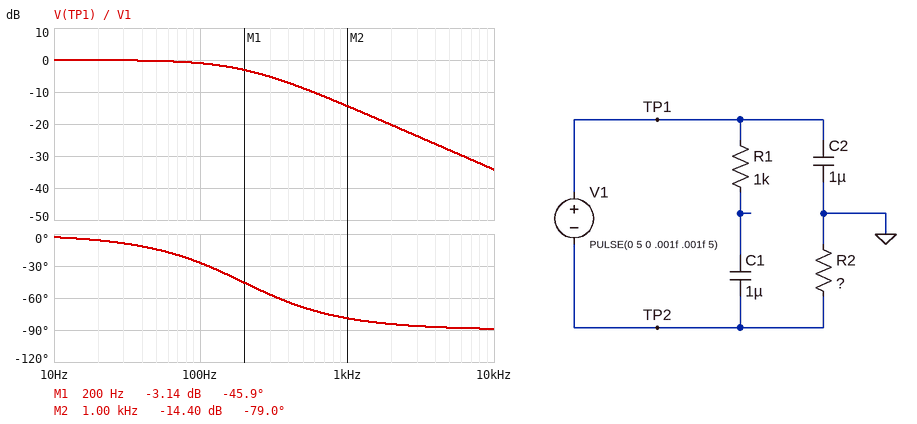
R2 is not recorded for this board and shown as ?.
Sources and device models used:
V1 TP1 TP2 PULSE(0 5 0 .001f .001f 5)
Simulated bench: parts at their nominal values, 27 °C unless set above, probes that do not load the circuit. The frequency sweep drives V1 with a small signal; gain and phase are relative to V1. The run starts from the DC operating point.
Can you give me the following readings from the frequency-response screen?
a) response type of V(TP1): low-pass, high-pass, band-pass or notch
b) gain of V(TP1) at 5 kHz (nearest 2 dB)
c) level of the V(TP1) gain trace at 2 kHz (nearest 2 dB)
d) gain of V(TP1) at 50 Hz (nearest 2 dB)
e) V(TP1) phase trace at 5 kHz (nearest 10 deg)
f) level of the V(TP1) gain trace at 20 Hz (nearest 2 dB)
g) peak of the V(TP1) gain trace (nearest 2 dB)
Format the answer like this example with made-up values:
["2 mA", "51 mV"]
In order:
["low-pass", "-28 dB", "-20 dB", "0 dB", "-90 deg", "0 dB", "0 dB"]
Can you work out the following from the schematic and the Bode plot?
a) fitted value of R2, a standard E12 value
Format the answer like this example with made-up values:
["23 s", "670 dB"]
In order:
["820 Ω"]
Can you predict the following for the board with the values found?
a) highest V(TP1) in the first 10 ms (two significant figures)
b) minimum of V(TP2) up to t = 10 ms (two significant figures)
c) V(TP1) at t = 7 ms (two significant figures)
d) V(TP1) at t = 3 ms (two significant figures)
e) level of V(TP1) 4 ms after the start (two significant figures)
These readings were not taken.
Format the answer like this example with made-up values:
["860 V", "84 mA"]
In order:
["5.0 V", "-5.0 V", "5.0 V", "4.9 V", "5.0 V"]
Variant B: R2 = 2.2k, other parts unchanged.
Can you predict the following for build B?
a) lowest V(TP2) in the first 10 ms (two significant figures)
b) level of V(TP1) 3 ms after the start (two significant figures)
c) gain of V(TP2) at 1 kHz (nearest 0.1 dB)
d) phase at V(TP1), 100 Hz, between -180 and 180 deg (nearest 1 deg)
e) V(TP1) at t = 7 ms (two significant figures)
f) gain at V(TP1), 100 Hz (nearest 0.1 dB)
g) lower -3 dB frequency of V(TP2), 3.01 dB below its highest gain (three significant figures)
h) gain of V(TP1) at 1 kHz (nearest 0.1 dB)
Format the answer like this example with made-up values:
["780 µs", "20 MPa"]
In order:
["-5.0 V", "3.7 V", "0 dB", "-54 deg", "4.8 V", "-4.6 dB", "72.3 Hz", "-22.8 dB"]
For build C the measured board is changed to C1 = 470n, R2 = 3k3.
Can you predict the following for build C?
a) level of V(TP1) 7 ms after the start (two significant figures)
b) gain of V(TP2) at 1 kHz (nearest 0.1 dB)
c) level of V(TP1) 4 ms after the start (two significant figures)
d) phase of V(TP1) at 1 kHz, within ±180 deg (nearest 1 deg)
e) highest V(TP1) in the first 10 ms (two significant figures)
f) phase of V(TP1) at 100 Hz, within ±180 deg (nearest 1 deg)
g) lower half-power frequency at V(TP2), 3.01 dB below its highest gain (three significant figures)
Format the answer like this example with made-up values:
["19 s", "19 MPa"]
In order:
["4.4 V", "0 dB", "3.5 V", "-87 deg", "4.8 V", "-64 deg", "48.2 Hz"]
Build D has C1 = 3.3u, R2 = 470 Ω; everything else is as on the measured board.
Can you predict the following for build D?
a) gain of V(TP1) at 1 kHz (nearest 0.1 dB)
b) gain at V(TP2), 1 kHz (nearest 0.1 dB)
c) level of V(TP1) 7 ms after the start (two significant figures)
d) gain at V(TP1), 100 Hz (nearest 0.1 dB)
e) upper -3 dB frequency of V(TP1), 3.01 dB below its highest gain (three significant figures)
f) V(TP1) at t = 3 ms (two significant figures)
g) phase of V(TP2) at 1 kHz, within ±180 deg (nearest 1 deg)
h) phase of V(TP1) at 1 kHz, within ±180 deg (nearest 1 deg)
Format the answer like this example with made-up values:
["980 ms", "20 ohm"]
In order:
["-9.9 dB", "-0.5 dB", "5.0 V", "-0.4 dB", "339 Hz", "5.0 V", "-161 deg", "-71 deg"]
